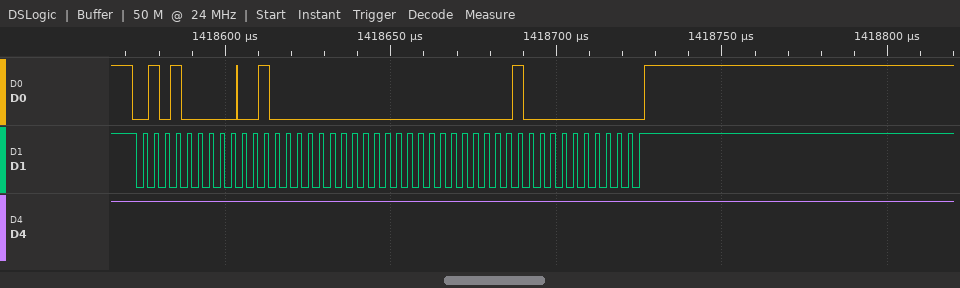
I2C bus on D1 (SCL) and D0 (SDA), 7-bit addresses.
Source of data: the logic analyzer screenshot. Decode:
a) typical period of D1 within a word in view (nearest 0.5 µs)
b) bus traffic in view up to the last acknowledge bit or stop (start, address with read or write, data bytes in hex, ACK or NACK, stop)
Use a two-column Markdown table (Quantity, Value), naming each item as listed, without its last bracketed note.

| Quantity | Value |
|---|---|
| typical period of D1 within a word in view | 3.5 µs |
| bus traffic in view up to the last acknowledge bit or stop | start, address 28 write ACK, 20 ACK, 00 ACK, 01 ACK, 00 ACK, stop |
